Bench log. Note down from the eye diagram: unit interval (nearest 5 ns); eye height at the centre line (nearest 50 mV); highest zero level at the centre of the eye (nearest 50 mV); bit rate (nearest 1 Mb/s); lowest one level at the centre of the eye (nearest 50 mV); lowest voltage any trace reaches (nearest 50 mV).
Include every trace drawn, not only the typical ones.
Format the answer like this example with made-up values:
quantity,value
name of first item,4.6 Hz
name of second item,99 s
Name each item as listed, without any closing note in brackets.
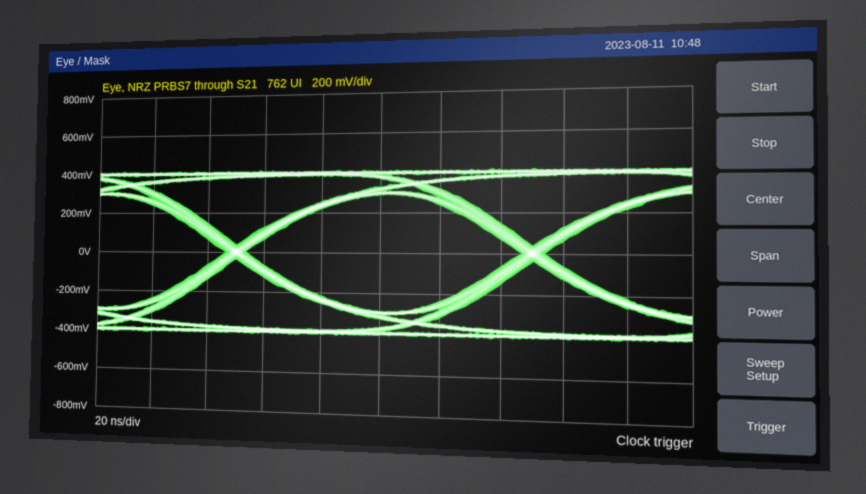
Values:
quantity,value
unit interval,100 ns
eye height at the centre line,600 mV
highest zero level at the centre of the eye,-300 mV
bit rate,10 Mb/s
lowest one level at the centre of the eye,300 mV
lowest voltage any trace reaches,-400 mV
